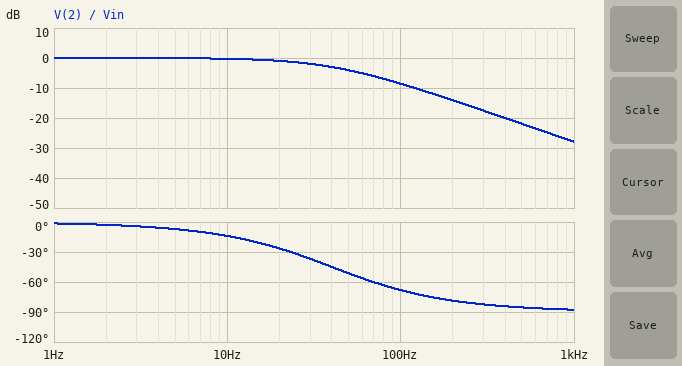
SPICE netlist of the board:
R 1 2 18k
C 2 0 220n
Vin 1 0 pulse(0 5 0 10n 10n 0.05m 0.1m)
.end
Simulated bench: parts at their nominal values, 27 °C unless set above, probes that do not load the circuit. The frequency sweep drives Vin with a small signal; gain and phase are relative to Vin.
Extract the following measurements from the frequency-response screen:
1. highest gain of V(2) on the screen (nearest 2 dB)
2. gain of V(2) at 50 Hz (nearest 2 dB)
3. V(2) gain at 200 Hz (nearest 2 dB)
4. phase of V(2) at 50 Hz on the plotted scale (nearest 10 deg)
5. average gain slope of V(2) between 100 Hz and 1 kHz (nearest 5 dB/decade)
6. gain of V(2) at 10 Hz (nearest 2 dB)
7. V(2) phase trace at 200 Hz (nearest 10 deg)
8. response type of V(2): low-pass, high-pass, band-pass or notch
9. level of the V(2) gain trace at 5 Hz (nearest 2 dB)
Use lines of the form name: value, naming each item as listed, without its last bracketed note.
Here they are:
highest gain of V(2) on the screen: 0 dB
gain of V(2) at 50 Hz: -4 dB
V(2) gain at 200 Hz: -14 dB
phase of V(2) at 50 Hz on the plotted scale: -50 deg
average gain slope of V(2) between 100 Hz and 1 kHz: -20 dB/decade
gain of V(2) at 10 Hz: 0 dB
V(2) phase trace at 200 Hz: -80 deg
response type of V(2): low-pass, high-pass, band-pass or notch: low-pass
level of the V(2) gain trace at 5 Hz: 0 dB
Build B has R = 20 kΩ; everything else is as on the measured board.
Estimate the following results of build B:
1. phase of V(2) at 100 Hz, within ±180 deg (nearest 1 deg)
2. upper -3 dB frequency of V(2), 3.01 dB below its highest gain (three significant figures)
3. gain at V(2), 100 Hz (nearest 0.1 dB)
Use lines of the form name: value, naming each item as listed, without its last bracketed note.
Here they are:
phase of V(2) at 100 Hz, within ±180 deg: -70 deg
upper -3 dB frequency of V(2), 3.01 dB below its highest gain: 36.2 Hz
gain at V(2), 100 Hz: -9.4 dB
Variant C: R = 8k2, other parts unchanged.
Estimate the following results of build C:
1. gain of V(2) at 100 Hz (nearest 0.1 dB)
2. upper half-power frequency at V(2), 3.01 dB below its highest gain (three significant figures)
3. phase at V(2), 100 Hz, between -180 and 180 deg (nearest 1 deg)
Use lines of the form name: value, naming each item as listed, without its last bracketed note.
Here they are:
gain of V(2) at 100 Hz: -3.6 dB
upper half-power frequency at V(2), 3.01 dB below its highest gain: 88.2 Hz
phase at V(2), 100 Hz, between -180 and 180 deg: -49 deg
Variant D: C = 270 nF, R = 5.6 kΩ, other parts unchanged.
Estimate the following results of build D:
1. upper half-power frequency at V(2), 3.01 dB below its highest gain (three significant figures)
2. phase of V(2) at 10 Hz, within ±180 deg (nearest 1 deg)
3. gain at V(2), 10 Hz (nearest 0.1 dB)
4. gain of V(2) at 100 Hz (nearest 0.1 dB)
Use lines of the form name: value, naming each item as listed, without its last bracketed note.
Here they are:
upper half-power frequency at V(2), 3.01 dB below its highest gain: 105 Hz
phase of V(2) at 10 Hz, within ±180 deg: -5 deg
gain at V(2), 10 Hz: 0 dB
gain of V(2) at 100 Hz: -2.8 dB
